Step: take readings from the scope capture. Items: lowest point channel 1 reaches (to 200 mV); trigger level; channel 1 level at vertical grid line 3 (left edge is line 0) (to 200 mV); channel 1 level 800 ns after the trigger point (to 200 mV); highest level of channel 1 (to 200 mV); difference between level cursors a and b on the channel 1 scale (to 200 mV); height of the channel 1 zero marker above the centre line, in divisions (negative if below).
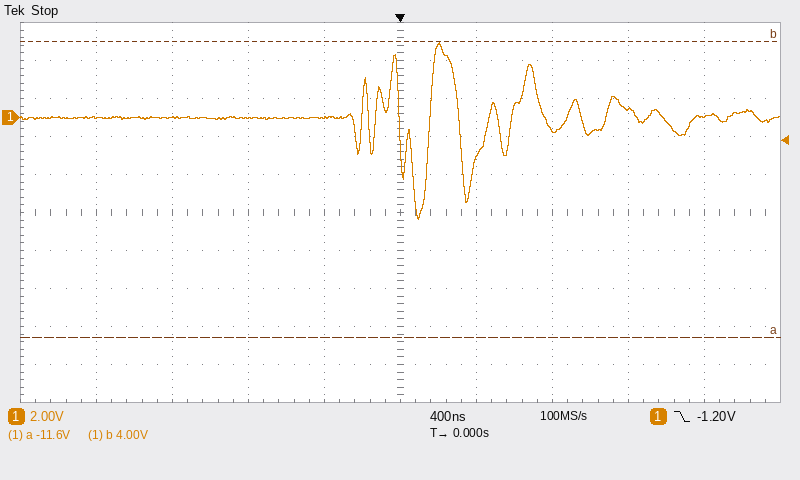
-5.4 V
-1.20 V
0.0 V
-600 mV
4.0 V
15.6 V
+2.5 div
